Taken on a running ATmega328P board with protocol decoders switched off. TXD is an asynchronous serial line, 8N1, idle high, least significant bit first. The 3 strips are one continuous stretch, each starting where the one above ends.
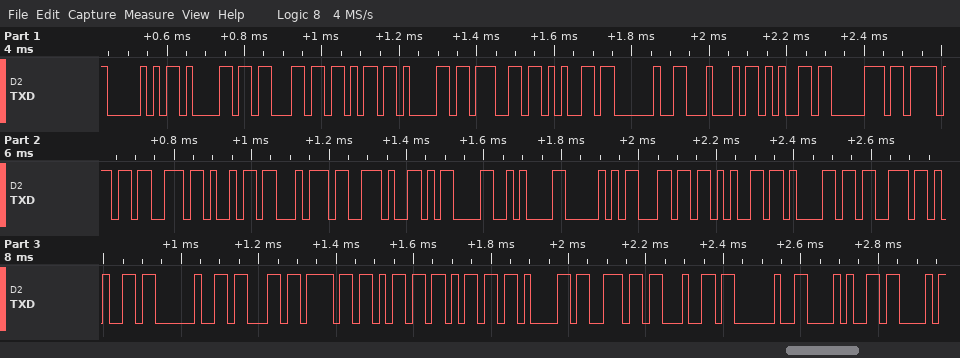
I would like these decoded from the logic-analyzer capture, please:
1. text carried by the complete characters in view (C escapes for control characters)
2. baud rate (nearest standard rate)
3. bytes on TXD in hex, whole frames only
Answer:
"Package Deposit.\r\nPlease command (C"
57600 baud
50 61 63 6B 61 67 65 20 44 65 70 6F 73 69 74 2E 0D 0A 50 6C 65 61 73 65 20 63 6F 6D 6D 61 6E 64 20 28 43
